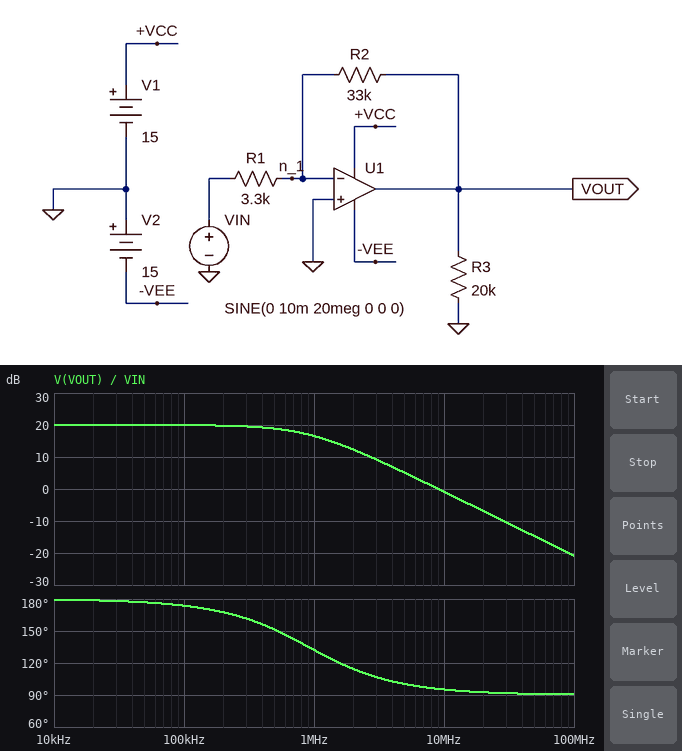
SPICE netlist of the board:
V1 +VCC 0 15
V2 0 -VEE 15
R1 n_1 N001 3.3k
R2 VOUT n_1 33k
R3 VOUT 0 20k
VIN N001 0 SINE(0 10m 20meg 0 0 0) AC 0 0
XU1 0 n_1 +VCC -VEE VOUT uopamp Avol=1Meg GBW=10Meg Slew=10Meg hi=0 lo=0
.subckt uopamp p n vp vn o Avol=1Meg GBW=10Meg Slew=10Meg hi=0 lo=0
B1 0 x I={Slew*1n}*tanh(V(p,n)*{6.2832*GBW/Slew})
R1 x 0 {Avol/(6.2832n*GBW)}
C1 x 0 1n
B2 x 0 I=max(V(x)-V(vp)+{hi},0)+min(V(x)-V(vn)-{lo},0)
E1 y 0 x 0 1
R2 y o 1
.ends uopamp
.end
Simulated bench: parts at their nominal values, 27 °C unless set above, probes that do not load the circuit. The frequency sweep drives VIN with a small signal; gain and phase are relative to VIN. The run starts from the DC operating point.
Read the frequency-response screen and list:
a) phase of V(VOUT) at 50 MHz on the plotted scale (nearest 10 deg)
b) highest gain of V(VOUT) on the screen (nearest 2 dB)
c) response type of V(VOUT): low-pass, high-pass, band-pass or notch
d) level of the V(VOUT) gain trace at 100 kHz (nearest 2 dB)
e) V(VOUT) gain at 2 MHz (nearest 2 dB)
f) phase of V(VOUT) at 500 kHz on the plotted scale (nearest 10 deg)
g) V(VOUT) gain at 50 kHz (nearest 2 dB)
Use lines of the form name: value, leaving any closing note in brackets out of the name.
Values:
phase of V(VOUT) at 50 MHz on the plotted scale: 90 deg
highest gain of V(VOUT) on the screen: 20 dB
response type of V(VOUT): low-pass, high-pass, band-pass or notch: low-pass
level of the V(VOUT) gain trace at 100 kHz: 20 dB
V(VOUT) gain at 2 MHz: 12 dB
phase of V(VOUT) at 500 kHz on the plotted scale: 150 deg
V(VOUT) gain at 50 kHz: 20 dB
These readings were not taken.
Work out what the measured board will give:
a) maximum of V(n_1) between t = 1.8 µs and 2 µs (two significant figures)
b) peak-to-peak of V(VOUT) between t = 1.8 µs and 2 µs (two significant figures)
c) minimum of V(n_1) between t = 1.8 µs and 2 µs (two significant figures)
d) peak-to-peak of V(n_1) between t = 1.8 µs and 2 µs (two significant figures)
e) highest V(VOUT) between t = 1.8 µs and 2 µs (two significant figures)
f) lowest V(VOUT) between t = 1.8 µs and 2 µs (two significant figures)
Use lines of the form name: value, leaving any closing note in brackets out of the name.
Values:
maximum of V(n_1) between t = 1.8 µs and 2 µs: 9.1 mV
peak-to-peak of V(VOUT) between t = 1.8 µs and 2 µs: 9.1 mV
minimum of V(n_1) between t = 1.8 µs and 2 µs: -9.1 mV
peak-to-peak of V(n_1) between t = 1.8 µs and 2 µs: 18 mV
highest V(VOUT) between t = 1.8 µs and 2 µs: 4.5 mV
lowest V(VOUT) between t = 1.8 µs and 2 µs: -4.5 mV
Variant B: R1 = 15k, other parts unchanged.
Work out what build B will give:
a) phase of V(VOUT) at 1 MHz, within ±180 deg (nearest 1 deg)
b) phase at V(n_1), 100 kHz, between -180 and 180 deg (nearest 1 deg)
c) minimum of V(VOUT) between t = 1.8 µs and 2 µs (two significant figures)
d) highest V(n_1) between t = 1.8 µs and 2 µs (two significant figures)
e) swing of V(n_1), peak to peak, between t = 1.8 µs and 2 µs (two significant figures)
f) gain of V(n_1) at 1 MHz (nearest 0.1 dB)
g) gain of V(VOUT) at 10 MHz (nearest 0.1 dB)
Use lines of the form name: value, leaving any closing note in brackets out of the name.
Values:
phase of V(VOUT) at 1 MHz, within ±180 deg: 162 deg
phase at V(n_1), 100 kHz, between -180 and 180 deg: 88 deg
minimum of V(VOUT) between t = 1.8 µs and 2 µs: -3.4 mV
highest V(n_1) between t = 1.8 µs and 2 µs: 6.8 mV
swing of V(n_1), peak to peak, between t = 1.8 µs and 2 µs: 14 mV
gain of V(n_1) at 1 MHz: -13.6 dB
gain of V(VOUT) at 10 MHz: -3.7 dB
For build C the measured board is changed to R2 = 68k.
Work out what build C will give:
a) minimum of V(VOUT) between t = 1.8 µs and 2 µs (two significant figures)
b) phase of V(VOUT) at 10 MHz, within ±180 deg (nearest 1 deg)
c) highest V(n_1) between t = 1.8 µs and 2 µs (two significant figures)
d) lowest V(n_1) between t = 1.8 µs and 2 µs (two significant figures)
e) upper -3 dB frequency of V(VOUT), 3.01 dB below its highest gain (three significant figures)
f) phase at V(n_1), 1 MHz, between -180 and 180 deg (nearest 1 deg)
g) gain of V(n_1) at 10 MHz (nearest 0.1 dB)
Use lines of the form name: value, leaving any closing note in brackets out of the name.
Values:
minimum of V(VOUT) between t = 1.8 µs and 2 µs: -4.8 mV
phase of V(VOUT) at 10 MHz, within ±180 deg: 93 deg
highest V(n_1) between t = 1.8 µs and 2 µs: 9.5 mV
lowest V(n_1) between t = 1.8 µs and 2 µs: -9.5 mV
upper -3 dB frequency of V(VOUT), 3.01 dB below its highest gain: 463 kHz
phase at V(n_1), 1 MHz, between -180 and 180 deg: 25 deg
gain of V(n_1) at 10 MHz: -0.4 dB
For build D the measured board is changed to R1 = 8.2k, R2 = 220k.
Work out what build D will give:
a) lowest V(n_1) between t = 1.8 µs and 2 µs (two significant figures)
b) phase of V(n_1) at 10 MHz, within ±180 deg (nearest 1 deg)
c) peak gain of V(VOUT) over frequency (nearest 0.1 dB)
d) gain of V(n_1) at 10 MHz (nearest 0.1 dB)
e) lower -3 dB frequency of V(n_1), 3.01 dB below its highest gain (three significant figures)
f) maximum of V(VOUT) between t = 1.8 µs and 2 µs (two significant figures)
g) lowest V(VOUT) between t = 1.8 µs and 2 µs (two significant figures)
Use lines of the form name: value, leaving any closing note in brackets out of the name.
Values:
lowest V(n_1) between t = 1.8 µs and 2 µs: -9.6 mV
phase of V(n_1) at 10 MHz, within ±180 deg: 2 deg
peak gain of V(VOUT) over frequency: 28.6 dB
gain of V(n_1) at 10 MHz: -0.3 dB
lower -3 dB frequency of V(n_1), 3.01 dB below its highest gain: 359 kHz
maximum of V(VOUT) between t = 1.8 µs and 2 µs: 4.8 mV
lowest V(VOUT) between t = 1.8 µs and 2 µs: -4.9 mV
